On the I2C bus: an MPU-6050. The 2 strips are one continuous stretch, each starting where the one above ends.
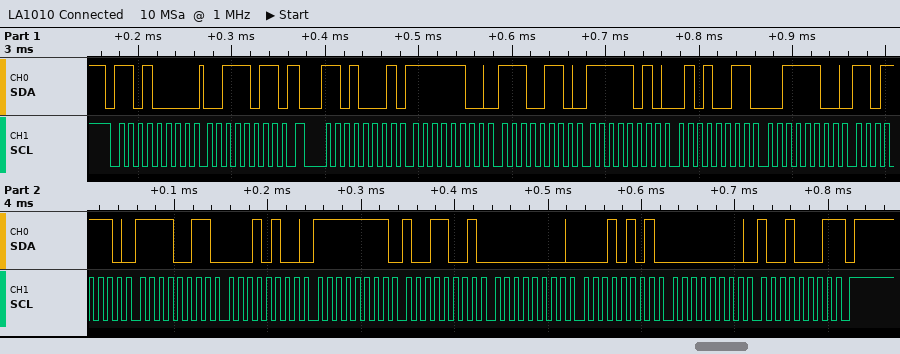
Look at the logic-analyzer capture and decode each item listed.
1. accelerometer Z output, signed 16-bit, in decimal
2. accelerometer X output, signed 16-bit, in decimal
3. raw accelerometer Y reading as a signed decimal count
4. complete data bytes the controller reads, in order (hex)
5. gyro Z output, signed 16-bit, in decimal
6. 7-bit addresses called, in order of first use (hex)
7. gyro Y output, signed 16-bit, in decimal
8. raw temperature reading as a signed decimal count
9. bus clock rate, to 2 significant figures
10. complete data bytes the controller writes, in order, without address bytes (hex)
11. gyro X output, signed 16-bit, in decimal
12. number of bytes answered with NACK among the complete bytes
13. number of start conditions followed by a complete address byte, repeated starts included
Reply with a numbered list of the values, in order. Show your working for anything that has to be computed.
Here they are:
1. 0x3CDE = 15582
2. 0xFCE6 = -794
3. 0xFA53 = -1453
4. FC E6 FA 53 3C DE F3 14 FF 99 00 15 00 91
5. 0x0091 = 145
6. 0x68
7. 0x0015 = 21
8. 0xF314 = -3308
9. 100 kHz
10. 3B
11. 0xFF99 = -103
12. 1
13. 2
